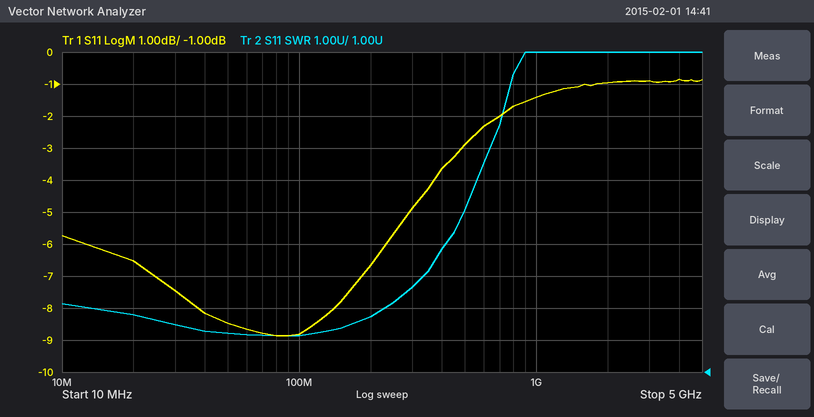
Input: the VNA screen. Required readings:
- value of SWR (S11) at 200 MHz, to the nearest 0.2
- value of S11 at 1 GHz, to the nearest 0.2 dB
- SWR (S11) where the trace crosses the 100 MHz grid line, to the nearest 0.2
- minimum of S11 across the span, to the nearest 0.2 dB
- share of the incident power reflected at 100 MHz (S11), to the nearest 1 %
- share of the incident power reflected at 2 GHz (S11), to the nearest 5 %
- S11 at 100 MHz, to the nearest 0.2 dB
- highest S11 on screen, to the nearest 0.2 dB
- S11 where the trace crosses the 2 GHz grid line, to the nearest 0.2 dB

2.8
-1.4 dB
2.2
-8.8 dB
13 %
80 %
-8.8 dB
-0.8 dB
-1.0 dB
